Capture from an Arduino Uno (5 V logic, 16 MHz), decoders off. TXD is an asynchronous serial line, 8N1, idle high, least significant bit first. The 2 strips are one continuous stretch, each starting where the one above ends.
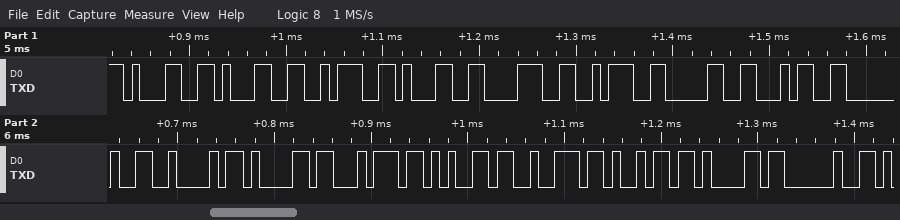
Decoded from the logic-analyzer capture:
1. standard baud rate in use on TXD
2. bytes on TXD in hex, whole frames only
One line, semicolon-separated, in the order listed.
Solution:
115200 baud; 0x31 0x31 0x3A 0x31 0x38 0x3A 0x30 0x34 0x20 0x42 0x61 0x74 0x65 0x72 0x69 0x61 0x20
